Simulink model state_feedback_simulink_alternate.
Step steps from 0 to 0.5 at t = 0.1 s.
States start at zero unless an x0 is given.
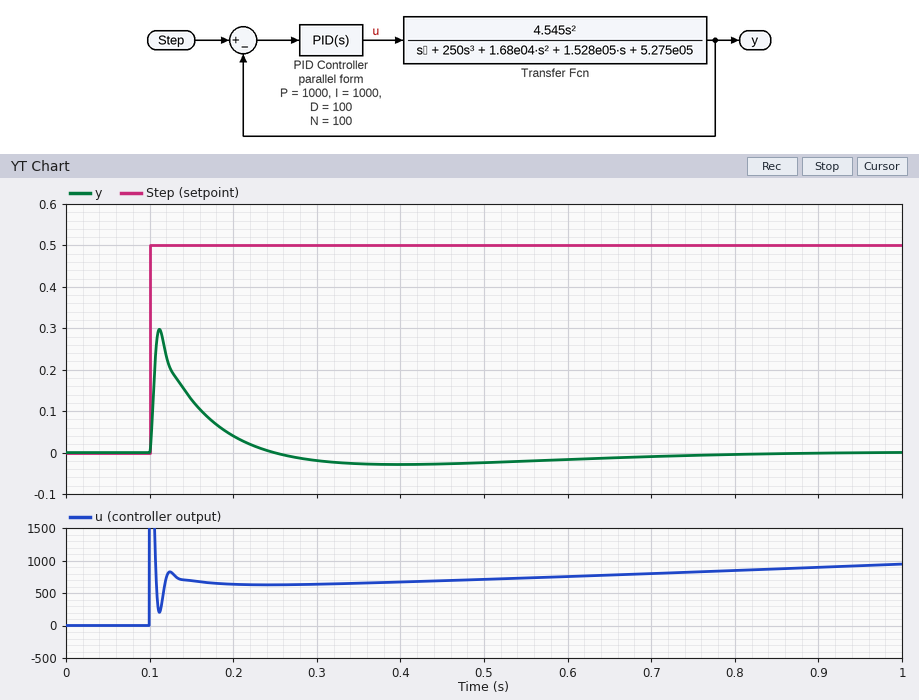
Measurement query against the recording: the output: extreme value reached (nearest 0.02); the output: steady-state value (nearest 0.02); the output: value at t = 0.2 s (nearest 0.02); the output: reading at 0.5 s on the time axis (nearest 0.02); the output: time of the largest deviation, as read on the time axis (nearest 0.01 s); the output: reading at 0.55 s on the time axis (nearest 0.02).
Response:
0.30
0.00
0.04
-0.02
0.11 s
-0.02
